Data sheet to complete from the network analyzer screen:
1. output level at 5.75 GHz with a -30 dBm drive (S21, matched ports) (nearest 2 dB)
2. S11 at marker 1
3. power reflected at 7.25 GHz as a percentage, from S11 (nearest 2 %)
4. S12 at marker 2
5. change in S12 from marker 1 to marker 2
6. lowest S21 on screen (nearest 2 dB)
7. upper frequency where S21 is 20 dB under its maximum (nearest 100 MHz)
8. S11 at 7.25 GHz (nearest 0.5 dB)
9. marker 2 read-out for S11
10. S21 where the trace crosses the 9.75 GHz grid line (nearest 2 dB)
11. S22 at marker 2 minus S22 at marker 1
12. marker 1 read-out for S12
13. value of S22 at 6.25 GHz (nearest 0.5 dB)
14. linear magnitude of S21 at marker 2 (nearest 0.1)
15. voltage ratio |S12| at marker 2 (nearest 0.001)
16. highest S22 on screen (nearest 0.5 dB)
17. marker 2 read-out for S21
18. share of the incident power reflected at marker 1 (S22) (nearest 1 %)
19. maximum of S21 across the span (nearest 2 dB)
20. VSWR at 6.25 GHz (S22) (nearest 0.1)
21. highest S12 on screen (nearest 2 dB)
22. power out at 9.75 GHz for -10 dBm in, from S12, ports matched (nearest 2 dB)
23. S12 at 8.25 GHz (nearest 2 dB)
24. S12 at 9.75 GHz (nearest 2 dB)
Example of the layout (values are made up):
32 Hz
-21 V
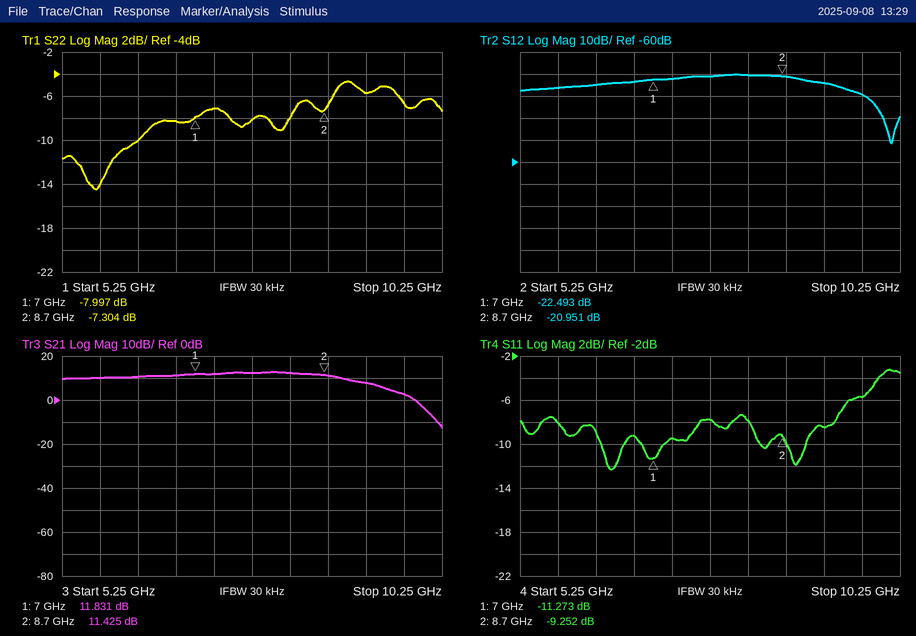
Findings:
-20 dBm
-11.273 dB
12 %
-20.951 dB
1.542 dB
-12 dB
10.1 GHz
-9.5 dB
-9.252 dB
2 dB
0.693 dB
-22.493 dB
-10.0 dB
3.7
0.090
-4.5 dB
11.425 dB
16 %
12 dB
1.9
-20 dB
-40 dBm
-20 dB
-30 dB
